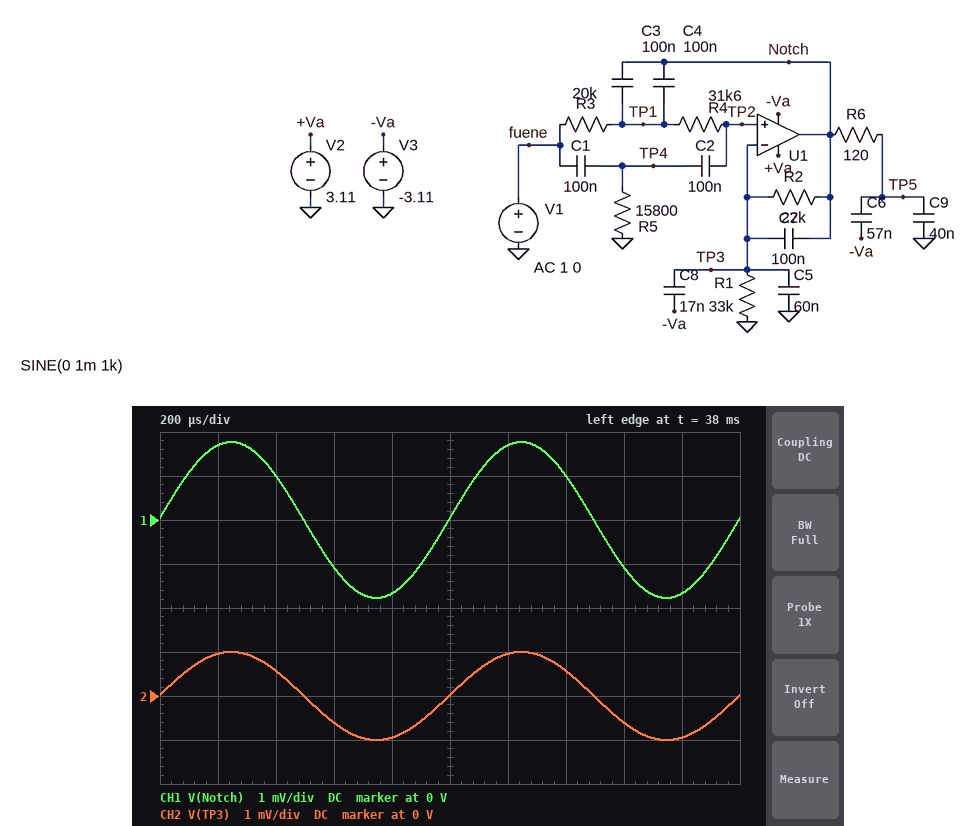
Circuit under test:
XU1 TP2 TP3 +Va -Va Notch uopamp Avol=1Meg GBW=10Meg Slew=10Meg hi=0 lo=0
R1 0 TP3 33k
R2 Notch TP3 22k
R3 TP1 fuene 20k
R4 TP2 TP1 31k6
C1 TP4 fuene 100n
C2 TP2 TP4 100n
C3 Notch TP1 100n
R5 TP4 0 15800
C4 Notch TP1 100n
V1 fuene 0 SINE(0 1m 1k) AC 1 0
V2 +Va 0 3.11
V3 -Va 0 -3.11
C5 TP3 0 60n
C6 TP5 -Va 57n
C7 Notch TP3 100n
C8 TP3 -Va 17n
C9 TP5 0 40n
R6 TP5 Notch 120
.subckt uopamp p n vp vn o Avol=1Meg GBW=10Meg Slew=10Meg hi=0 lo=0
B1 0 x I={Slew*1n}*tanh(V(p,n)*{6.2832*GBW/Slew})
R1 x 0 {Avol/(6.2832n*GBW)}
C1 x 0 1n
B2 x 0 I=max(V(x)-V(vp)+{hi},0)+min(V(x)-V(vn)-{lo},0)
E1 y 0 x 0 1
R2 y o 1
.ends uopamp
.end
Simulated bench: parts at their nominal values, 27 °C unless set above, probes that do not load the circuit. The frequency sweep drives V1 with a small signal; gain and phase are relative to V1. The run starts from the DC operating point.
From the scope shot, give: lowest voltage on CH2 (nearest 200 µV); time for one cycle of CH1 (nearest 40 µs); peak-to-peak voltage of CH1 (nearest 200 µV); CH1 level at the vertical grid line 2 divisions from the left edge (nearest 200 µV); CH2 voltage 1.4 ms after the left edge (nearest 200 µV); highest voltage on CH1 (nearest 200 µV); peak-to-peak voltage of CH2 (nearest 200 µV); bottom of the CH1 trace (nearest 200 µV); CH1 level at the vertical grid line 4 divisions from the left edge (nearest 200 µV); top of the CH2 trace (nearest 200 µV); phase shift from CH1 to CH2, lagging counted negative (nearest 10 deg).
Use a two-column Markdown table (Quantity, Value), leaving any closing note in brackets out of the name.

| Quantity | Value |
|---|---|
| lowest voltage on CH2 | -1.0 mV |
| time for one cycle of CH1 | 1.00 ms |
| peak-to-peak voltage of CH1 | 3.6 mV |
| CH1 level at the vertical grid line 2 divisions from the left edge | 1.0 mV |
| CH2 voltage 1.4 ms after the left edge | 600 µV |
| highest voltage on CH1 | 1.8 mV |
| peak-to-peak voltage of CH2 | 2.0 mV |
| bottom of the CH1 trace | -1.8 mV |
| CH1 level at the vertical grid line 4 divisions from the left edge | -1.6 mV |
| top of the CH2 trace | 1.0 mV |
| phase shift from CH1 to CH2, lagging counted negative | 0 deg |
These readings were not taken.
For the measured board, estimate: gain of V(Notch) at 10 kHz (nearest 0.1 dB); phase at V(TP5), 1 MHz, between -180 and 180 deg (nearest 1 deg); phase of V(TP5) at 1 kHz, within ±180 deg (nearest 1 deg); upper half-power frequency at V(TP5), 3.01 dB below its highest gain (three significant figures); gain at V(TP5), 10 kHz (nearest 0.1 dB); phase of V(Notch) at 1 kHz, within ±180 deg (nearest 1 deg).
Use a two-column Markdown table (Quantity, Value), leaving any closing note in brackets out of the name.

| Quantity | Value |
|---|---|
| gain of V(Notch) at 10 kHz | 5.0 dB |
| phase at V(TP5), 1 MHz, between -180 and 180 deg | -100 deg |
| phase of V(TP5) at 1 kHz, within ±180 deg | -3 deg |
| upper half-power frequency at V(TP5), 3.01 dB below its highest gain | 12.5 kHz |
| gain at V(TP5), 10 kHz | 3.1 dB |
| phase of V(Notch) at 1 kHz, within ±180 deg | 2 deg |
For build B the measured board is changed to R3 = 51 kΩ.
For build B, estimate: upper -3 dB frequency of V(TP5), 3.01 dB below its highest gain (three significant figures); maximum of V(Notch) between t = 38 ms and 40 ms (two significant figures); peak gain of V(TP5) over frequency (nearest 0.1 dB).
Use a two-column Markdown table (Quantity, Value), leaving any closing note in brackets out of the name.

| Quantity | Value |
|---|---|
| upper -3 dB frequency of V(TP5), 3.01 dB below its highest gain | 13.7 kHz |
| maximum of V(Notch) between t = 38 ms and 40 ms | 1.8 mV |
| peak gain of V(TP5) over frequency | 4.9 dB |
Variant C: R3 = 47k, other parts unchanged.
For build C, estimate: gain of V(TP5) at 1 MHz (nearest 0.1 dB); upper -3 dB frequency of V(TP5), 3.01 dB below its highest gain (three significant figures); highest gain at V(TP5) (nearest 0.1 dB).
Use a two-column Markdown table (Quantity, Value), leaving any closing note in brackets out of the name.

| Quantity | Value |
|---|---|
| gain of V(TP5) at 1 MHz | -32.0 dB |
| upper -3 dB frequency of V(TP5), 3.01 dB below its highest gain | 13.7 kHz |
| highest gain at V(TP5) | 4.9 dB |
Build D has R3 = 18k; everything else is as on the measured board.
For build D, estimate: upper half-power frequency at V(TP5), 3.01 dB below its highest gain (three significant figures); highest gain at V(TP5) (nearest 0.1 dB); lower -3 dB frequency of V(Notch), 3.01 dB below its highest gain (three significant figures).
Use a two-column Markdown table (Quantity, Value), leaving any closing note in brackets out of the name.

| Quantity | Value |
|---|---|
| upper half-power frequency at V(TP5), 3.01 dB below its highest gain | 12.3 kHz |
| highest gain at V(TP5) | 5.4 dB |
| lower -3 dB frequency of V(Notch), 3.01 dB below its highest gain | 97.9 Hz |
